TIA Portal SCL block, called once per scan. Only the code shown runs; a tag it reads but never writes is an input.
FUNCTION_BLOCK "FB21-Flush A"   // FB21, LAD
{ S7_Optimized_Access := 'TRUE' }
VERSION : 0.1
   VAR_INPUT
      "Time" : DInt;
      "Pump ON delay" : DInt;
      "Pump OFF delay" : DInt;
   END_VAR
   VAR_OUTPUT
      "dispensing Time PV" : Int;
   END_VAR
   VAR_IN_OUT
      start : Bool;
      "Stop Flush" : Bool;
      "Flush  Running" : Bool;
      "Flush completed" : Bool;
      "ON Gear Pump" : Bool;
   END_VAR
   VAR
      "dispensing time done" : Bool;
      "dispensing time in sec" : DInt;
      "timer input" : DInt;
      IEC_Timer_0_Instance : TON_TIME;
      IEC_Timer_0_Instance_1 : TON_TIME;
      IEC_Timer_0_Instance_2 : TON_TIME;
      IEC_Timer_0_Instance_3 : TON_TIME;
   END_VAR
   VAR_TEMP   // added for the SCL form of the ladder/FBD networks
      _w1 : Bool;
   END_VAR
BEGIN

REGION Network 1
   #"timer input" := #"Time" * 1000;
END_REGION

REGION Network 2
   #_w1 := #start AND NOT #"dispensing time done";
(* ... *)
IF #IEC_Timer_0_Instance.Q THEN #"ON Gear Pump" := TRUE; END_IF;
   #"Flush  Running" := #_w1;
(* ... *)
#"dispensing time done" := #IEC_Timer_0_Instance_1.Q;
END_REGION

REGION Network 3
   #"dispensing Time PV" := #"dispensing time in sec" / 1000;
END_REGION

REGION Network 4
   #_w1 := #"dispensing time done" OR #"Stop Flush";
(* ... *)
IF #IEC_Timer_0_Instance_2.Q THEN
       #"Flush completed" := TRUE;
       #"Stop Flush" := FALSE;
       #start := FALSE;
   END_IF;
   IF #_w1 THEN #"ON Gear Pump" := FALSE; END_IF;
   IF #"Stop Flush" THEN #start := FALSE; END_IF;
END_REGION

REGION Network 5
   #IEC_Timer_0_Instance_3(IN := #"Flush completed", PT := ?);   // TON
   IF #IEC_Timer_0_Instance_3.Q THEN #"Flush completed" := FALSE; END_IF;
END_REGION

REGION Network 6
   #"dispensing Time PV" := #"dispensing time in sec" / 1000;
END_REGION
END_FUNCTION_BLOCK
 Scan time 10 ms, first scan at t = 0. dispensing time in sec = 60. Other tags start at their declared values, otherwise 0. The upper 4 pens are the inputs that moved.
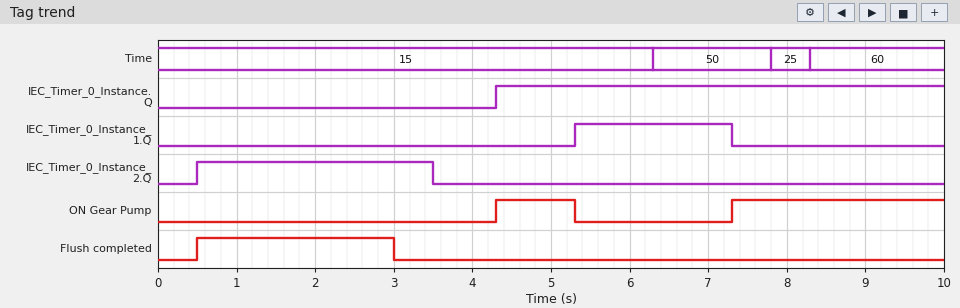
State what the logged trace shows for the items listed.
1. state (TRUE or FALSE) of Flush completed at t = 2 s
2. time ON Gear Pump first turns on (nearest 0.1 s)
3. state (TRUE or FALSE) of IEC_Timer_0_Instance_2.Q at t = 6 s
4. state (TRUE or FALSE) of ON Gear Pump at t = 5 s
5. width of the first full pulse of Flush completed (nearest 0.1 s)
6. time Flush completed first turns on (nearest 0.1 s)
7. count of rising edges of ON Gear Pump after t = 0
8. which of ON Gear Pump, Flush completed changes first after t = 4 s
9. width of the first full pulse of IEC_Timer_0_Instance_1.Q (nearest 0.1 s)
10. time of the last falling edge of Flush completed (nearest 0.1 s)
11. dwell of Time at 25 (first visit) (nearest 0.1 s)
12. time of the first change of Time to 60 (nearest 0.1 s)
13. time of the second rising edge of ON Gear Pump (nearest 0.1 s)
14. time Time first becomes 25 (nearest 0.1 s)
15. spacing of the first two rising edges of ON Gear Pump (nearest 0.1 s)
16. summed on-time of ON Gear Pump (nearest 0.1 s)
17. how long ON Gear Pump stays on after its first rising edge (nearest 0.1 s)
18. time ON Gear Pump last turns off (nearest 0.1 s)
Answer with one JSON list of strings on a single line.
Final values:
["TRUE", "4.3 s", "FALSE", "TRUE", "2.5 s", "0.5 s", "2", "ON Gear Pump", "2.0 s", "3.0 s", "0.5 s", "8.3 s", "7.3 s", "7.8 s", "3.0 s", "3.7 s", "1.0 s", "5.3 s"]
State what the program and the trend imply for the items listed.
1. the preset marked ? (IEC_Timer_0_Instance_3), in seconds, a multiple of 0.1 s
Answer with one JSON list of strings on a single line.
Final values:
["2.5 s"]
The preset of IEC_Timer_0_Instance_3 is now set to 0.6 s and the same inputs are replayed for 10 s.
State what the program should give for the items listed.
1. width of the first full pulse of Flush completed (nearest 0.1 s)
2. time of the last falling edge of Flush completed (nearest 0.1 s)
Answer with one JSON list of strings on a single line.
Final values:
["0.6 s", "1.1 s"]
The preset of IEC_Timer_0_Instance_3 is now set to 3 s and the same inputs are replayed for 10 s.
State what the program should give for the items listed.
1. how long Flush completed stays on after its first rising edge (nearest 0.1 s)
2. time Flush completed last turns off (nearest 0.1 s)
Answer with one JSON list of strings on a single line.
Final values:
["3.0 s", "3.5 s"]
